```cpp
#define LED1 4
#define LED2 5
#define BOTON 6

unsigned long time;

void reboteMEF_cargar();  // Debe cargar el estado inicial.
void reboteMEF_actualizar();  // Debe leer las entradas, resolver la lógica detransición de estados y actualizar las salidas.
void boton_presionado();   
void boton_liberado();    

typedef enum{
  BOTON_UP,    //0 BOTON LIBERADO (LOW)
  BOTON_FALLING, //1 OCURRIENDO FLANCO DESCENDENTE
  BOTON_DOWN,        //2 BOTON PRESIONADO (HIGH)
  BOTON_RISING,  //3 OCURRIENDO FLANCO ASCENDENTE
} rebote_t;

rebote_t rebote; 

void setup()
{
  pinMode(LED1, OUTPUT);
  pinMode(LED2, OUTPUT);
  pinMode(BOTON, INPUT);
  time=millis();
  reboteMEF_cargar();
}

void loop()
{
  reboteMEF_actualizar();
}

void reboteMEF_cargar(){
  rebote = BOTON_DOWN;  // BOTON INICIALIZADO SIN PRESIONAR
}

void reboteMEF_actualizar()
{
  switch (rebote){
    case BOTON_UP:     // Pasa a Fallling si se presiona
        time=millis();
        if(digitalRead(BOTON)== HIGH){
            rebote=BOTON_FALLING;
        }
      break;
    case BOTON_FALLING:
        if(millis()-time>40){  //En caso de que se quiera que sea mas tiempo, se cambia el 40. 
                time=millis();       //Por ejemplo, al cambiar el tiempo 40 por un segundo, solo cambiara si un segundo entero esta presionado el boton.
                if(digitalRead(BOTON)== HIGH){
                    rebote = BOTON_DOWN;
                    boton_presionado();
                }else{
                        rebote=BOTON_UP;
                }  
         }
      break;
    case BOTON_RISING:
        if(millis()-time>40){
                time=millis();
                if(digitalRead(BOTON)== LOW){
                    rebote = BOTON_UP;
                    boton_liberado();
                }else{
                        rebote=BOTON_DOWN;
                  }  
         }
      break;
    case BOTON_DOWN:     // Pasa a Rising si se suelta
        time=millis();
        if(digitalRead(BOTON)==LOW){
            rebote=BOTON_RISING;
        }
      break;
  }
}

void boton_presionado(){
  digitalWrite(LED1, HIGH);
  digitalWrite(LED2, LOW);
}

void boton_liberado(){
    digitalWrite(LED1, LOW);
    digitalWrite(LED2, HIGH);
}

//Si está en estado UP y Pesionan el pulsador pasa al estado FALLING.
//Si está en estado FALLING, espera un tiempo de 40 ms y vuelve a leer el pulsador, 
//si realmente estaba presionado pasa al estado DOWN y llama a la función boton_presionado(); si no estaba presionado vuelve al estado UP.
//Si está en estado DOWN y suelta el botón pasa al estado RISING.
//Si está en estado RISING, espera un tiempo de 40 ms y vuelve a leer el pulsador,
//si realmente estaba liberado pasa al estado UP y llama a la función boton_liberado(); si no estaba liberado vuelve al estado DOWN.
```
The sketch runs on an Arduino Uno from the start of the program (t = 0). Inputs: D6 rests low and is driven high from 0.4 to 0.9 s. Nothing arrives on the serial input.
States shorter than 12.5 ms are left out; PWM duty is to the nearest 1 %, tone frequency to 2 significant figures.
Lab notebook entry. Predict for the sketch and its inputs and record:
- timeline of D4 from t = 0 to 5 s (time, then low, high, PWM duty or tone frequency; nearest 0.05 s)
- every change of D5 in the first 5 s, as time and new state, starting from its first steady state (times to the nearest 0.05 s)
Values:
0 s low; 0.45 s high; 0.95 s low
0 s low; 0.05 s high; 0.45 s low; 0.95 s high
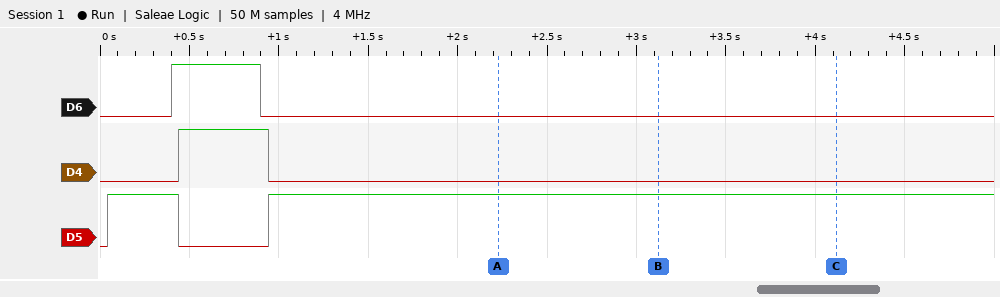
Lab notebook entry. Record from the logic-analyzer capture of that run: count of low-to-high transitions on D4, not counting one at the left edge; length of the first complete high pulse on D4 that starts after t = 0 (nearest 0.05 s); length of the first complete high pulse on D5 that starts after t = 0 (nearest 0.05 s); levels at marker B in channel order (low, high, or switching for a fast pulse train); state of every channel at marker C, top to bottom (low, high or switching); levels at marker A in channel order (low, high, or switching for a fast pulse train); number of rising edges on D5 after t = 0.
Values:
1
0.50 s
0.40 s
D6 low, D4 low, D5 high
D6 low, D4 low, D5 high
D6 low, D4 low, D5 high
2
